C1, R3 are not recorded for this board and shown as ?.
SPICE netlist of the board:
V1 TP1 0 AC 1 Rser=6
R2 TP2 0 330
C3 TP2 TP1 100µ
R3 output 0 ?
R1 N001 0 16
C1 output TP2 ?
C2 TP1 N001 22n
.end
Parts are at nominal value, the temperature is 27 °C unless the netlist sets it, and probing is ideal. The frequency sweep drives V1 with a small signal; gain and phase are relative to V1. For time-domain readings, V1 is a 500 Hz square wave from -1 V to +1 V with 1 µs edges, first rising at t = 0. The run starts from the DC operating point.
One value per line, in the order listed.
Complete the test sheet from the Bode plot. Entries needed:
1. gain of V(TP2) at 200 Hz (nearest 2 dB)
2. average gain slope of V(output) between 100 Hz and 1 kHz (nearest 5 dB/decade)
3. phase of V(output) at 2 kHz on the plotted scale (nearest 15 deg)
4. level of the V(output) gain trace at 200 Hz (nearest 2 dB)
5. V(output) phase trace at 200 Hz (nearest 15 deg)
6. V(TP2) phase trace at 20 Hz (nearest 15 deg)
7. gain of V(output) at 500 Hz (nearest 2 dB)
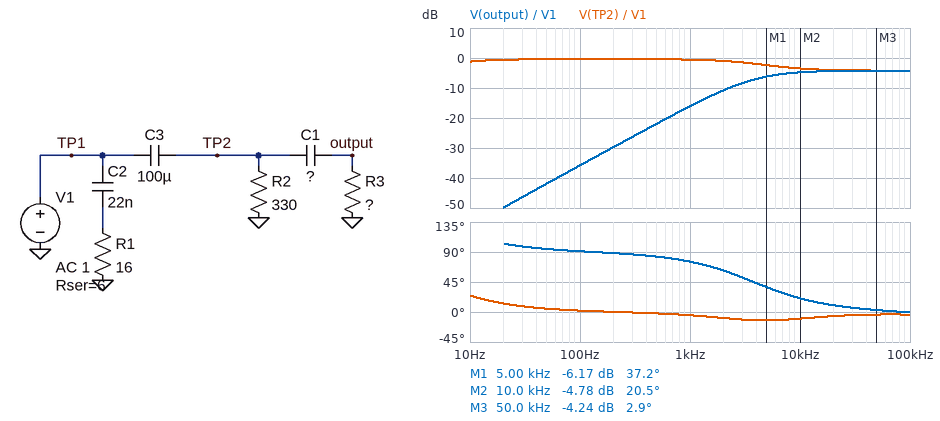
0 dB
20 dB/decade
60 deg
-30 dB
90 deg
15 deg
-22 dB
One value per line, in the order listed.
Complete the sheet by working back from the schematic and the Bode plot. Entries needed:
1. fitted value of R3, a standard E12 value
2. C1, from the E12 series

10 Ω
2.7 µF
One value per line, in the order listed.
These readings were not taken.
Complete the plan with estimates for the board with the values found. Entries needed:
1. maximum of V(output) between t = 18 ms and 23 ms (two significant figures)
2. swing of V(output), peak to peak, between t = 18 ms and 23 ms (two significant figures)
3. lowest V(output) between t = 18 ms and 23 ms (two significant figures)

1.2 V
2.4 V
-1.2 V
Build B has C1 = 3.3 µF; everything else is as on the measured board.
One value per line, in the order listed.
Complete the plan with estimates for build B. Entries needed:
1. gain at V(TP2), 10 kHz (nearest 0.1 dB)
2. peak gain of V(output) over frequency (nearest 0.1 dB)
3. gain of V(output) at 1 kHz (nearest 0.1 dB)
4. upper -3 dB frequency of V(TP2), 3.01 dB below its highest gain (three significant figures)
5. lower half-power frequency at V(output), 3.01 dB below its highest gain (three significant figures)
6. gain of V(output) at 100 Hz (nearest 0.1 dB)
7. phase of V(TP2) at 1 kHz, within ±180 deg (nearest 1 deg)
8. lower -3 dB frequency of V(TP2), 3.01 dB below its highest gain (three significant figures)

-3.7 dB
-4.2 dB
-14.5 dB
7.92 kHz
3.10 kHz
-34.1 dB
-6 deg
4.58 Hz
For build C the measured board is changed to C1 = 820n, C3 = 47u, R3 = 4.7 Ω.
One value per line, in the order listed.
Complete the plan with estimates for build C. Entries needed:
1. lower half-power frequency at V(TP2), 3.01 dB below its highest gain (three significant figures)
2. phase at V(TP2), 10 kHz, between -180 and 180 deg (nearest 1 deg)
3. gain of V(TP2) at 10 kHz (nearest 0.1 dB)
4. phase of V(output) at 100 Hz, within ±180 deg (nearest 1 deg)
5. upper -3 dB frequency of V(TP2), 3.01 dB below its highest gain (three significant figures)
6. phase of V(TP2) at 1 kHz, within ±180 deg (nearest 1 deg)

9.90 Hz
-15 deg
-1.2 dB
95 deg
23.8 kHz
-1 deg
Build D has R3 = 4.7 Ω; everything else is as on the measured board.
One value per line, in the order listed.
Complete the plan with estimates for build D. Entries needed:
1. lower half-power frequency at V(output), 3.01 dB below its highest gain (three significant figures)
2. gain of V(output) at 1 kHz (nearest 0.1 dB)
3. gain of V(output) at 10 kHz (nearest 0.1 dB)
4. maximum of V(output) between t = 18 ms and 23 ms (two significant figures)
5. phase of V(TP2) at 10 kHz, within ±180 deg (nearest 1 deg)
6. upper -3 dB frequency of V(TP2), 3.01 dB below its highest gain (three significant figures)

5.61 kHz
-22.5 dB
-8.5 dB
830 mV
-22 deg
7.44 kHz
